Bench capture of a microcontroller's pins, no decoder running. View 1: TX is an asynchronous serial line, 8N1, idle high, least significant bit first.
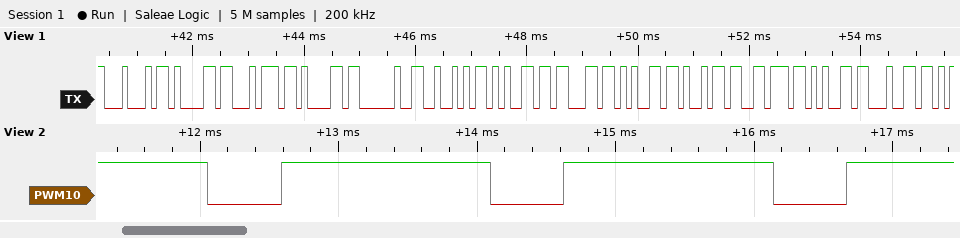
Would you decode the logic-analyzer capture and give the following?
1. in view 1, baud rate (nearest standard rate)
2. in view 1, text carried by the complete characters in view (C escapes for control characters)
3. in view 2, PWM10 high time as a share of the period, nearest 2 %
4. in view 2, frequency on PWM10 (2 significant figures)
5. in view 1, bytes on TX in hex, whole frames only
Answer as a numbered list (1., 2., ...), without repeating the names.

1. 9600 baud
2. "Data Received"
3. 74 %
4. 490 Hz
5. 44 61 74 61 20 52 65 63 65 69 76 65 64
